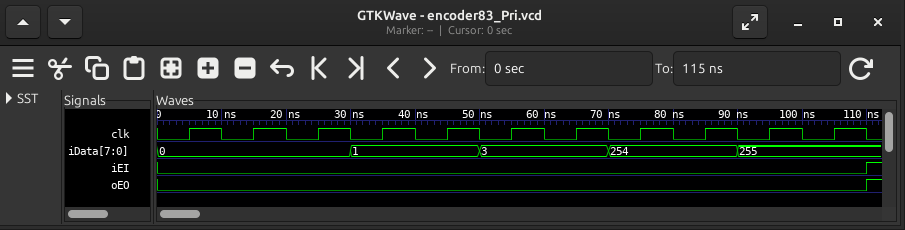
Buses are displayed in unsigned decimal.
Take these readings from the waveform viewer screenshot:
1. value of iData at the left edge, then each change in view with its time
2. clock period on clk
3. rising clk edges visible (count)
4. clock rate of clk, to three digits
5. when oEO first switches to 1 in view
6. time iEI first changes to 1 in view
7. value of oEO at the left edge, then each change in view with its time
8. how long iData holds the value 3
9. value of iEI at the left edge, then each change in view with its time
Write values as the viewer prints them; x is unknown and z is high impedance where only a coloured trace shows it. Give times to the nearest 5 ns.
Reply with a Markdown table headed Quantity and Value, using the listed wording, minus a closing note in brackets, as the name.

| Quantity | Value |
|---|---|
| value of iData at the left edge, then each change in view with its time | 0, 1 at 30 ns, 3 at 50 ns, 254 at 70 ns, 255 at 90 ns |
| clock period on clk | 10 ns |
| rising clk edges visible | 11 |
| clock rate of clk, to three digits | 100 MHz |
| when oEO first switches to 1 in view | 110 ns |
| time iEI first changes to 1 in view | 110 ns |
| value of oEO at the left edge, then each change in view with its time | 0, 1 at 110 ns |
| how long iData holds the value 3 | 20 ns |
| value of iEI at the left edge, then each change in view with its time | 0, 1 at 110 ns |
